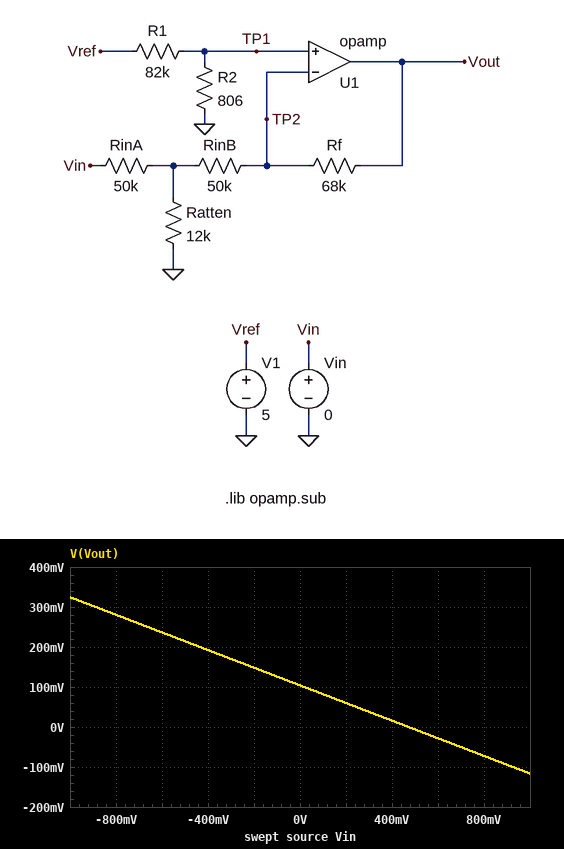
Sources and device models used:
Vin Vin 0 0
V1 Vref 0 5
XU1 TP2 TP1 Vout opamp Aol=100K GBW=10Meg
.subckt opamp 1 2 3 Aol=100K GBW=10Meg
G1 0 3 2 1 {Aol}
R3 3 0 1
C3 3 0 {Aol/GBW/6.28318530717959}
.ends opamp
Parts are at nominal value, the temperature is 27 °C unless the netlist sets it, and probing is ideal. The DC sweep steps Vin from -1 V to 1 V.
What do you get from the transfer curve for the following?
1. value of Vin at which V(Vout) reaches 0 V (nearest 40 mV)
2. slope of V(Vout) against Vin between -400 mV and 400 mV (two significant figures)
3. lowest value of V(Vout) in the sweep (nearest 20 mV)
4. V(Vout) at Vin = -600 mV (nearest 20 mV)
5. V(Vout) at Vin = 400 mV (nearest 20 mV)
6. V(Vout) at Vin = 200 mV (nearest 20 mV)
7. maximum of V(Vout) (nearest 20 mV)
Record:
480 mV
-0.22 V/V
-120 mV
240 mV
20 mV
60 mV
320 mV
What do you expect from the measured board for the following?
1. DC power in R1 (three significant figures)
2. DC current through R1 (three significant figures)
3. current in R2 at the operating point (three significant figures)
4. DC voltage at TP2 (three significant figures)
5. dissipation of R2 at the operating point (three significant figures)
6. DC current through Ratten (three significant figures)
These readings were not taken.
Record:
299 µW
60.4 µA
60.4 µA
48.7 mV
2.94 µW
658 nA
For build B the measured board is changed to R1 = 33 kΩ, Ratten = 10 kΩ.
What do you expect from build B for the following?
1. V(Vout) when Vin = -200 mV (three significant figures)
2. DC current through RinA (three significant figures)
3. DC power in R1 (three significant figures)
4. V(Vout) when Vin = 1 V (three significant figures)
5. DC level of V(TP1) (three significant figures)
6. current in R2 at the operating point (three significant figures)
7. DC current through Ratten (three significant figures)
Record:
297 mV
341 nA
722 µW
63.9 mV
119 mV
148 µA
1.70 µA
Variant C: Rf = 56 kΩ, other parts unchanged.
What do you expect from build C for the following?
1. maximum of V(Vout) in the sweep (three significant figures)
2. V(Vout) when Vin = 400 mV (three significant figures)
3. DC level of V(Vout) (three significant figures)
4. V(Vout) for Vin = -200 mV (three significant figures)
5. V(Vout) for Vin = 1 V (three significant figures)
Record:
276 mV
21.7 mV
94.3 mV
131 mV
-87.3 mV
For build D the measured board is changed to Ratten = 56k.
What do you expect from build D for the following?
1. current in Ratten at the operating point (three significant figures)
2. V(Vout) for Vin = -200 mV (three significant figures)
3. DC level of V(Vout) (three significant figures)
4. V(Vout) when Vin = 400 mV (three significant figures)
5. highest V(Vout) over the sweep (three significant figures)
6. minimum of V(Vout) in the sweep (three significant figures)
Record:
300 nA
186 mV
92.0 mV
-96.1 mV
562 mV
-378 mV
